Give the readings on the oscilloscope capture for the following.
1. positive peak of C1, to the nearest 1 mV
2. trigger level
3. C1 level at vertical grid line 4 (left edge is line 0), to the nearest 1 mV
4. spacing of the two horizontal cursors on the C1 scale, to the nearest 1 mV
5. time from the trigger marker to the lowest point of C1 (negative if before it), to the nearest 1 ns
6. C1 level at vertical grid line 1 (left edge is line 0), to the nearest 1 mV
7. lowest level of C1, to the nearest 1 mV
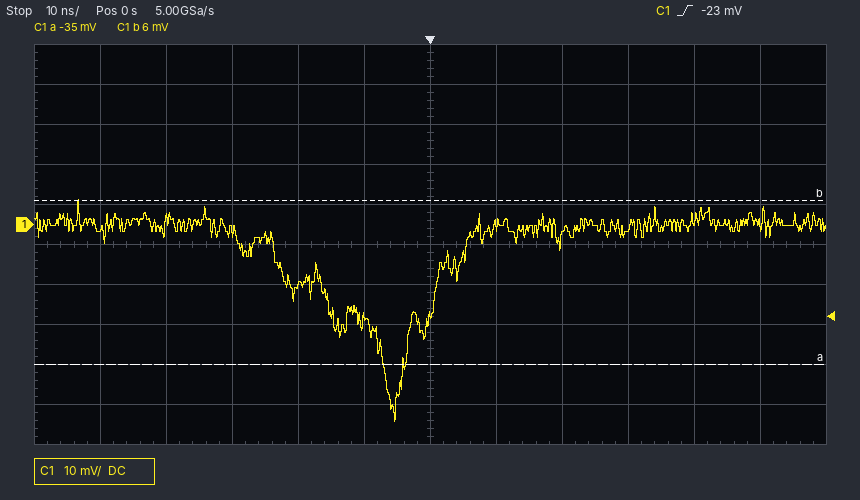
6 mV
-23 mV
-15 mV
41 mV
-5 ns
-1 mV
-49 mV
